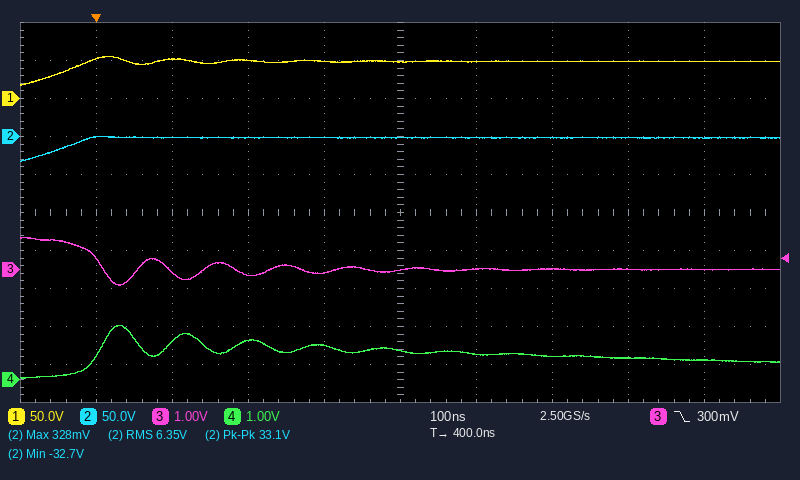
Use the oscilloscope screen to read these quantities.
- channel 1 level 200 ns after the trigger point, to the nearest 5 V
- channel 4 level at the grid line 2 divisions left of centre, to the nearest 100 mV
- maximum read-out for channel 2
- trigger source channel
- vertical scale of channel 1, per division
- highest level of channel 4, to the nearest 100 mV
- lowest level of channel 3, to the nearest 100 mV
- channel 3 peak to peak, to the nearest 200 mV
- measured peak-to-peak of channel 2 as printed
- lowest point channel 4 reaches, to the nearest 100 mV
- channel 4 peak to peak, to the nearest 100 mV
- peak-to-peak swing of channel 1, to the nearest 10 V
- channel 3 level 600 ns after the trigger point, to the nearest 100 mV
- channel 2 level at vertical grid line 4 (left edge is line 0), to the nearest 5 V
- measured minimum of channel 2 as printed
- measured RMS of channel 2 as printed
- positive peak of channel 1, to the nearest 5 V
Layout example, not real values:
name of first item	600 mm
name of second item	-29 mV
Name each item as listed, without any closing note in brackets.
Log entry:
channel 1 level 200 ns after the trigger point, to the nearest 5 V	50 V
channel 4 level at the grid line 2 divisions left of centre, to the nearest 100 mV	1.0 V
maximum read-out for channel 2	328 mV
trigger source channel	channel 3
vertical scale of channel 1, per division	50 V
highest level of channel 4, to the nearest 100 mV	1.4 V
lowest level of channel 3, to the nearest 100 mV	-400 mV
channel 3 peak to peak, to the nearest 200 mV	1.2 V
measured peak-to-peak of channel 2 as printed	33.1 V
lowest point channel 4 reaches, to the nearest 100 mV	0.0 V
channel 4 peak to peak, to the nearest 100 mV	1.4 V
peak-to-peak swing of channel 1, to the nearest 10 V	40 V
channel 3 level 600 ns after the trigger point, to the nearest 100 mV	0.0 V
channel 2 level at vertical grid line 4 (left edge is line 0), to the nearest 5 V	0 V
measured minimum of channel 2 as printed	-32.7 V
measured RMS of channel 2 as printed	6.35 V
positive peak of channel 1, to the nearest 5 V	55 V
